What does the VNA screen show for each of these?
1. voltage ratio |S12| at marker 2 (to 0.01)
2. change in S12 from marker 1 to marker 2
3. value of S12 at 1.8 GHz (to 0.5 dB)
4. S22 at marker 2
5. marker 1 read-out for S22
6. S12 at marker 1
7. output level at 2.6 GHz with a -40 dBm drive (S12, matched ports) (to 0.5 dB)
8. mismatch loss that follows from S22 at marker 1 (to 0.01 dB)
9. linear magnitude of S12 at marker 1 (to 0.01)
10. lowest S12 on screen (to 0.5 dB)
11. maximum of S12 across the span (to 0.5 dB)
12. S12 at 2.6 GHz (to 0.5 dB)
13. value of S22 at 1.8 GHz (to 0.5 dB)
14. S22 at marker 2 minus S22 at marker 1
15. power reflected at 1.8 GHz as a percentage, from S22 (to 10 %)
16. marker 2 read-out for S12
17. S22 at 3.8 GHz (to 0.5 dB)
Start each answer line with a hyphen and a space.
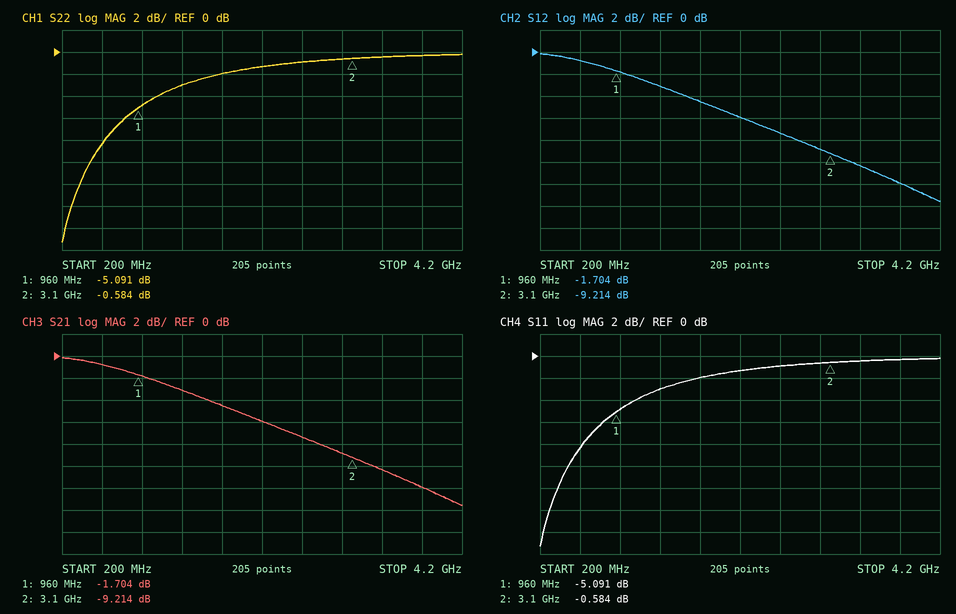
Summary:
- 0.35
- -7.510 dB
- -4.5 dB
- -0.584 dB
- -5.091 dB
- -1.704 dB
- -47.5 dBm
- 1.61 dB
- 0.82
- -13.5 dB
- 0.0 dB
- -7.5 dB
- -2.0 dB
- 4.507 dB
- 60 %
- -9.214 dB
- -0.5 dB
